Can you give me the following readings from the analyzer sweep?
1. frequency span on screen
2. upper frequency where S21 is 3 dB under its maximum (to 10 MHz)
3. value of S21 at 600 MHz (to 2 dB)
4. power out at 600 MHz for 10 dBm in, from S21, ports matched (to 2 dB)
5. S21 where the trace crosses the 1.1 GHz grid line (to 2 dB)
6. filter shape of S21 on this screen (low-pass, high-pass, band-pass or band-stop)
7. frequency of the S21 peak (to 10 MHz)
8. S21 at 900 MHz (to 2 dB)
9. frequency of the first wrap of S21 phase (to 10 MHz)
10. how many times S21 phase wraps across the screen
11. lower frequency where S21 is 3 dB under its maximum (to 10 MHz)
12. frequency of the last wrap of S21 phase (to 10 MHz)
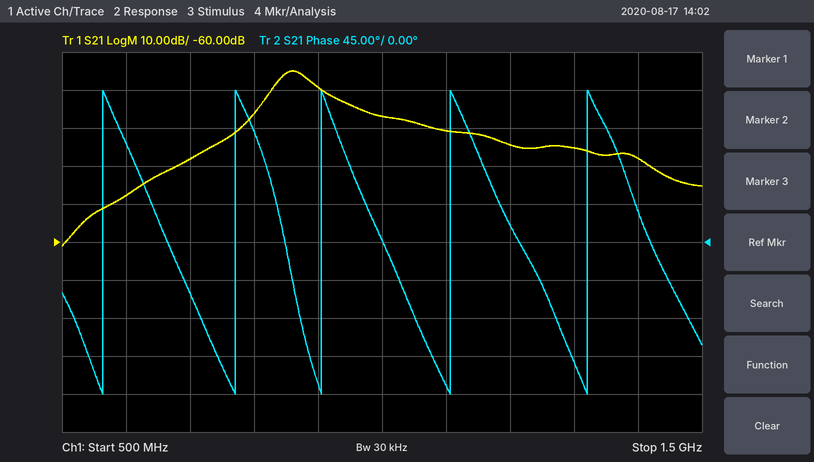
1 GHz
890 MHz
-48 dB
-38 dBm
-30 dB
band-pass
860 MHz
-20 dB
560 MHz
5
840 MHz
1.32 GHz
